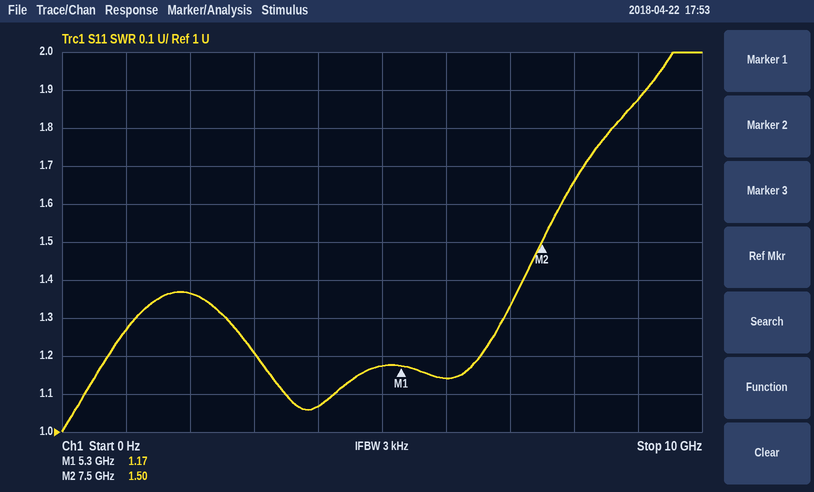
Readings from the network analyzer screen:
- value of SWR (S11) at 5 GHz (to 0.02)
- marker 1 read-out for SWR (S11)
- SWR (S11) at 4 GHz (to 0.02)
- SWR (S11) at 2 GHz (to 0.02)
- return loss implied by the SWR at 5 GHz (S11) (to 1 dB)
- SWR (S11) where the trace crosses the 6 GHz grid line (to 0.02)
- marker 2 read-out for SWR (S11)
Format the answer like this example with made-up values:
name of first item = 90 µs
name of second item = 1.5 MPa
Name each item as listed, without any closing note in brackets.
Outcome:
value of SWR (S11) at 5 GHz = 1.18
marker 1 read-out for SWR = 1.17
SWR (S11) at 4 GHz = 1.06
SWR (S11) at 2 GHz = 1.36
return loss implied by the SWR at 5 GHz (S11) = 22 dB
SWR (S11) where the trace crosses the 6 GHz grid line = 1.14
marker 2 read-out for SWR = 1.50
